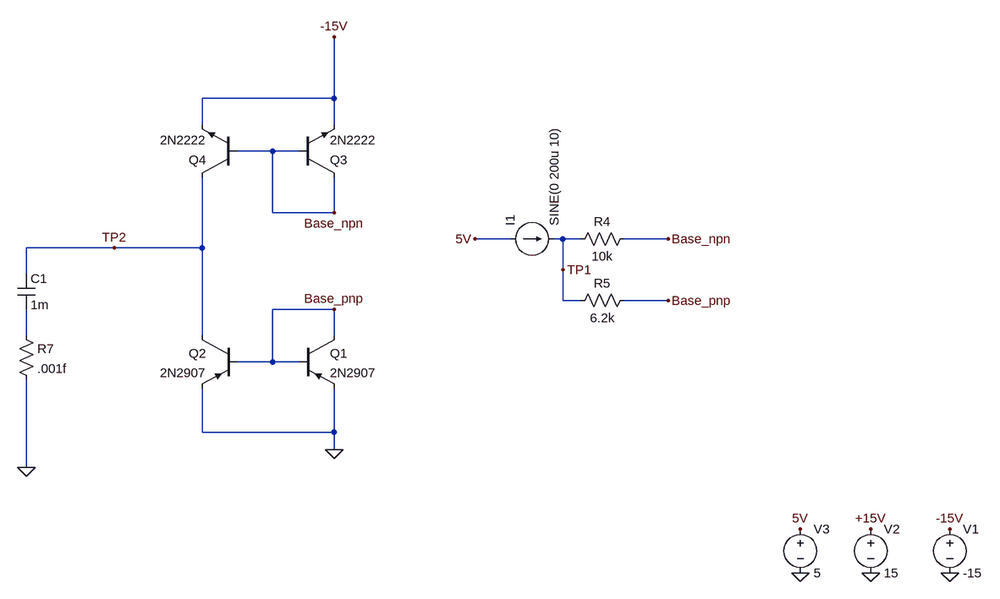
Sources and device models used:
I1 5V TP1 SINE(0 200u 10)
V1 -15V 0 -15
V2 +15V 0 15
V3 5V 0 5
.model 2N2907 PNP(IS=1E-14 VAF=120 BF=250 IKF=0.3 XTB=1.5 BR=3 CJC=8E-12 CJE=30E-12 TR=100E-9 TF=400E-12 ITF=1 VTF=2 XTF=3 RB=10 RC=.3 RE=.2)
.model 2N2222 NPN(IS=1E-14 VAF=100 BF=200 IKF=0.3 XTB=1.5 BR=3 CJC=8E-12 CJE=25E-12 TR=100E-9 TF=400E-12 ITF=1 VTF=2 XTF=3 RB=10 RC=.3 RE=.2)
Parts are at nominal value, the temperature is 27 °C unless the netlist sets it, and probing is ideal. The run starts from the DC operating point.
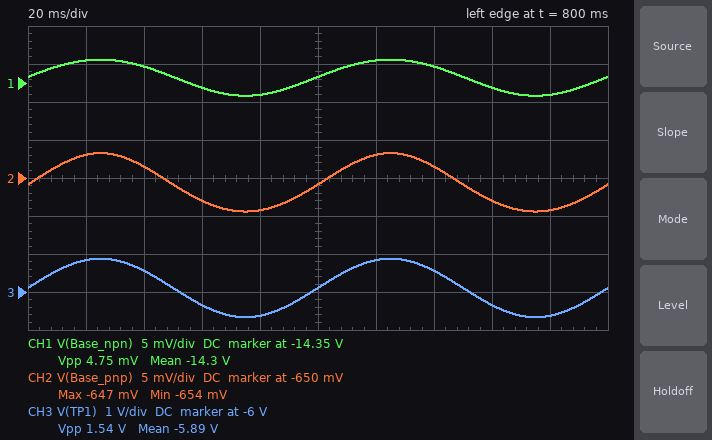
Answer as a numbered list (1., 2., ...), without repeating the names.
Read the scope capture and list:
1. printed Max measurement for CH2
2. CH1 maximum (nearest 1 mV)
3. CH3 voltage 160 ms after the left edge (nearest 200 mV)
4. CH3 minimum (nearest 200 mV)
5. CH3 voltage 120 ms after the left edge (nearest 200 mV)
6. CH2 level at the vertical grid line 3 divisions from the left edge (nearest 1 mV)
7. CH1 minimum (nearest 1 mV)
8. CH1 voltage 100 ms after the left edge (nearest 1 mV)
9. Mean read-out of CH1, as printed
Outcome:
1. -647 mV
2. -14.347 V
3. -6.4 V
4. -6.6 V
5. -5.2 V
6. -653 mV
7. -14.352 V
8. -14.349 V
9. -14.3 V
